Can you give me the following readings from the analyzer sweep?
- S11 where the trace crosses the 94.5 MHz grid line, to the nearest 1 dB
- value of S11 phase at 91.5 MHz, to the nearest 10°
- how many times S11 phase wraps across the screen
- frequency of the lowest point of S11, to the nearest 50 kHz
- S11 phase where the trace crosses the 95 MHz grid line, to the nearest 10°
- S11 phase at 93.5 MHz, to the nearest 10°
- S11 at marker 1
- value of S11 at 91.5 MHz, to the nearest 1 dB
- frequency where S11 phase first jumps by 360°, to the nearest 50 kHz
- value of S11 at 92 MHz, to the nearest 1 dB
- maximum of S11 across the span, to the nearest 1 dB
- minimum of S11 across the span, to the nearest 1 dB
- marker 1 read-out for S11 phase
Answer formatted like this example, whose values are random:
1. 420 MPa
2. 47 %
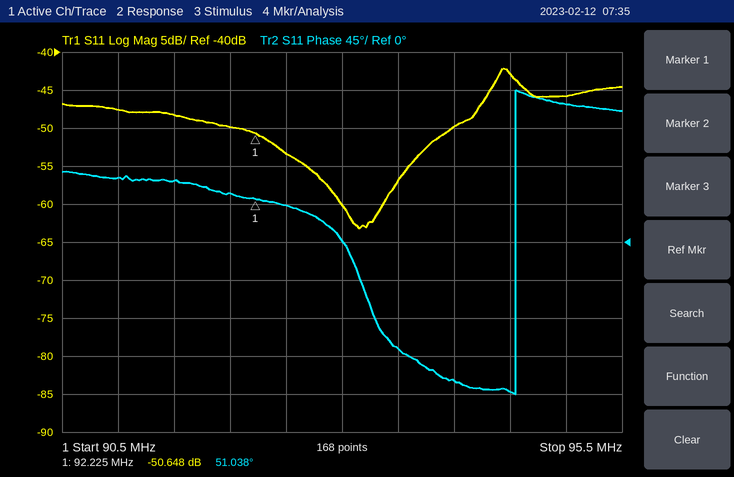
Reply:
1. -43 dB
2. 70°
3. 1
4. 93.15 MHz
5. 160°
6. -130°
7. -50.648 dB
8. -48 dB
9. 94.55 MHz
10. -50 dB
11. -42 dB
12. -63 dB
13. 51.038°
